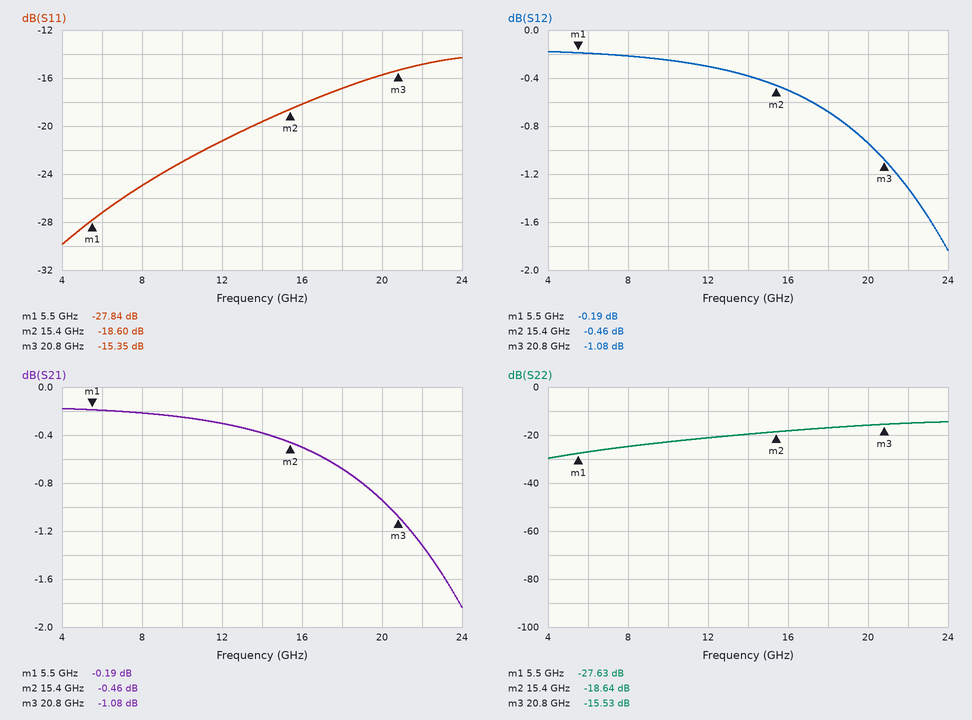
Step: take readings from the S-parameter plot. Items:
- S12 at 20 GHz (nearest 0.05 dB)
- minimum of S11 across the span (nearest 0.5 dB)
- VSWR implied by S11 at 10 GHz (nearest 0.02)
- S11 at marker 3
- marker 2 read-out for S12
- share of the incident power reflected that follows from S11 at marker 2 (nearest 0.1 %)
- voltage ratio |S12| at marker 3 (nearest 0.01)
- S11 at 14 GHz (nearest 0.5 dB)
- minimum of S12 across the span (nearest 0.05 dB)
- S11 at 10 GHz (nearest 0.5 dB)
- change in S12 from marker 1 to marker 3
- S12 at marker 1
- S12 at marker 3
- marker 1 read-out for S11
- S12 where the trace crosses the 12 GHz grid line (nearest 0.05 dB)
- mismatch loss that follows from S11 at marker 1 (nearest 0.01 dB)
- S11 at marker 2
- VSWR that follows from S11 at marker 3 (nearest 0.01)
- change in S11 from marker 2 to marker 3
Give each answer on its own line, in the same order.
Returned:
-0.95 dB
-30.0 dB
1.16
-15.35 dB
-0.46 dB
1.4 %
0.88
-19.5 dB
-1.85 dB
-23.0 dB
-0.89 dB
-0.19 dB
-1.08 dB
-27.84 dB
-0.30 dB
0.01 dB
-18.60 dB
1.41
3.25 dB
